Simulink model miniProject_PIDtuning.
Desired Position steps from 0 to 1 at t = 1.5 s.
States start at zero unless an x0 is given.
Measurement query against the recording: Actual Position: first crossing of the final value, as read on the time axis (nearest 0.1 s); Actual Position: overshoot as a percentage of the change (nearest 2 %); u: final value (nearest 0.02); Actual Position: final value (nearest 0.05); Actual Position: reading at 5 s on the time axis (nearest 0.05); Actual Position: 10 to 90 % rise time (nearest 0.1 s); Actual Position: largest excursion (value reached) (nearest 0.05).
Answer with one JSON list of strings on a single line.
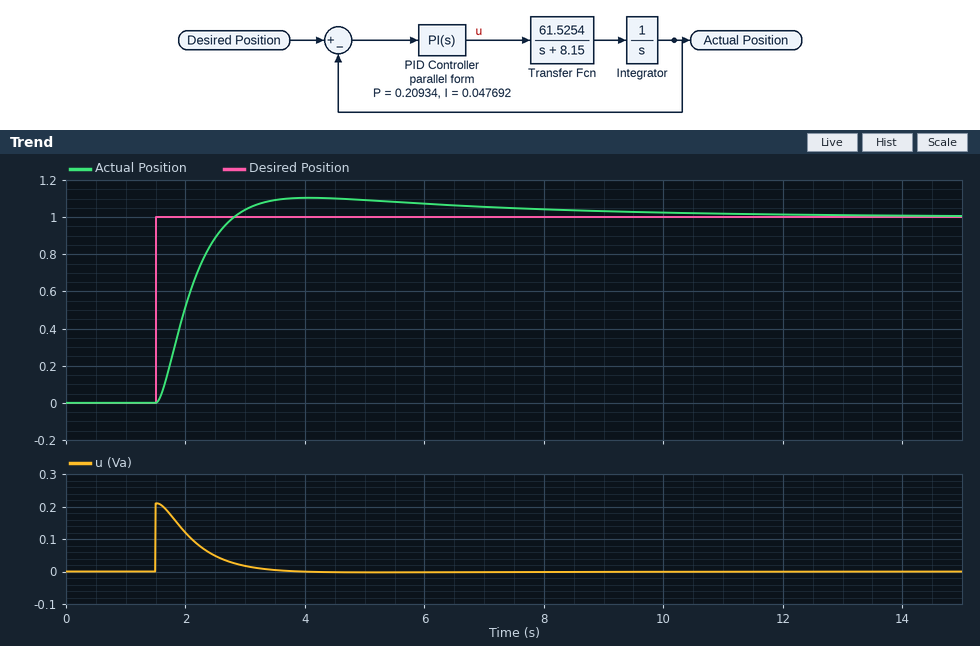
["2.8 s", "10 %", "0.00", "1.00", "1.10", "0.9 s", "1.10"]
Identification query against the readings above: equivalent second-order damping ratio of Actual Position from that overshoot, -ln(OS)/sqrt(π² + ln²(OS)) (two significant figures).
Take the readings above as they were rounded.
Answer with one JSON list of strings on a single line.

["0.59"]
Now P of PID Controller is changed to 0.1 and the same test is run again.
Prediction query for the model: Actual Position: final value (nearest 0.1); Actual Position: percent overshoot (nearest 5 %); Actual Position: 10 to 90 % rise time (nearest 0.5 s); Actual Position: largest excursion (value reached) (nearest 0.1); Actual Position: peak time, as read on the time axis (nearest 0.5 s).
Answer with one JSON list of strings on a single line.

["1.0", "25 %", "1.5 s", "1.3", "5.0 s"]
